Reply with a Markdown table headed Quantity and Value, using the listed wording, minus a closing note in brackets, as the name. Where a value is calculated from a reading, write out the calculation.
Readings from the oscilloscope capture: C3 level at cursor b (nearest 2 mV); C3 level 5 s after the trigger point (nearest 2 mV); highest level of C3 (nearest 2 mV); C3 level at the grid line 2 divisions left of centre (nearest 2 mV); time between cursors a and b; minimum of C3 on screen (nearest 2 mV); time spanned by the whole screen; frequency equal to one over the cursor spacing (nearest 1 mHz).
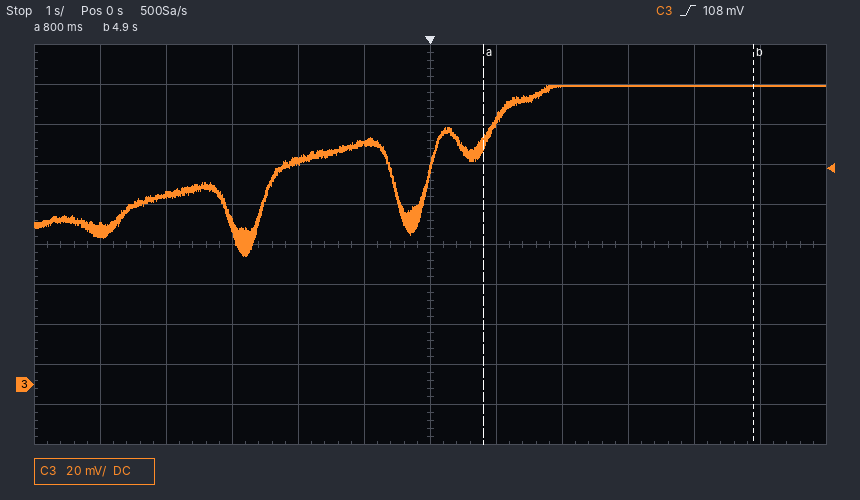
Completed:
| Quantity | Value |
|---|---|
| C3 level at cursor b | 150 mV |
| C3 level 5 s after the trigger point | 150 mV |
| highest level of C3 | 150 mV |
| C3 level at the grid line 2 divisions left of centre | 112 mV |
| time between cursors a and b | 4.9 s − (800 ms) = 4.1 s |
| minimum of C3 on screen | 64 mV |
| time spanned by the whole screen | 12 s |
| frequency equal to one over the cursor spacing | 1 / 4.1 s ≈ 244 mHz |
